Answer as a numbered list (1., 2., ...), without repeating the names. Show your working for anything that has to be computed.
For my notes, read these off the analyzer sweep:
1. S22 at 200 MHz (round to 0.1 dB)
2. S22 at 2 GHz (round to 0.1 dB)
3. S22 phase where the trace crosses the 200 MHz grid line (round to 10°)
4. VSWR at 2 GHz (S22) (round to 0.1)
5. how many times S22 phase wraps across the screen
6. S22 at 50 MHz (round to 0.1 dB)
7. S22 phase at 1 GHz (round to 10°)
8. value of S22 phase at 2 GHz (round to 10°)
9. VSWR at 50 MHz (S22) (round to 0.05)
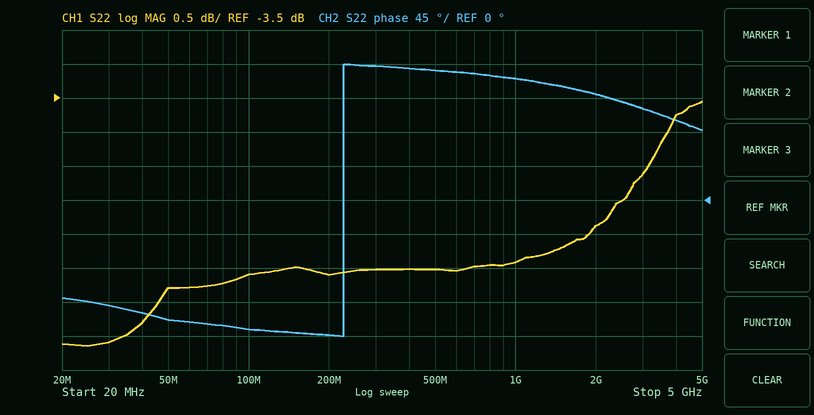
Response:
1. -6.1 dB
2. -5.4 dB
3. -180°
4. |Γ| = 10^(-5.4/20) = 0.5370; VSWR = (1 + 0.5370)/(1 − 0.5370) ≈ 3.3
5. 1
6. -6.3 dB
7. 160°
8. 140°
9. |Γ| = 10^(-6.3/20) = 0.4842; VSWR = (1 + 0.4842)/(1 − 0.4842) ≈ 2.88, so 2.90 to the nearest 0.05
